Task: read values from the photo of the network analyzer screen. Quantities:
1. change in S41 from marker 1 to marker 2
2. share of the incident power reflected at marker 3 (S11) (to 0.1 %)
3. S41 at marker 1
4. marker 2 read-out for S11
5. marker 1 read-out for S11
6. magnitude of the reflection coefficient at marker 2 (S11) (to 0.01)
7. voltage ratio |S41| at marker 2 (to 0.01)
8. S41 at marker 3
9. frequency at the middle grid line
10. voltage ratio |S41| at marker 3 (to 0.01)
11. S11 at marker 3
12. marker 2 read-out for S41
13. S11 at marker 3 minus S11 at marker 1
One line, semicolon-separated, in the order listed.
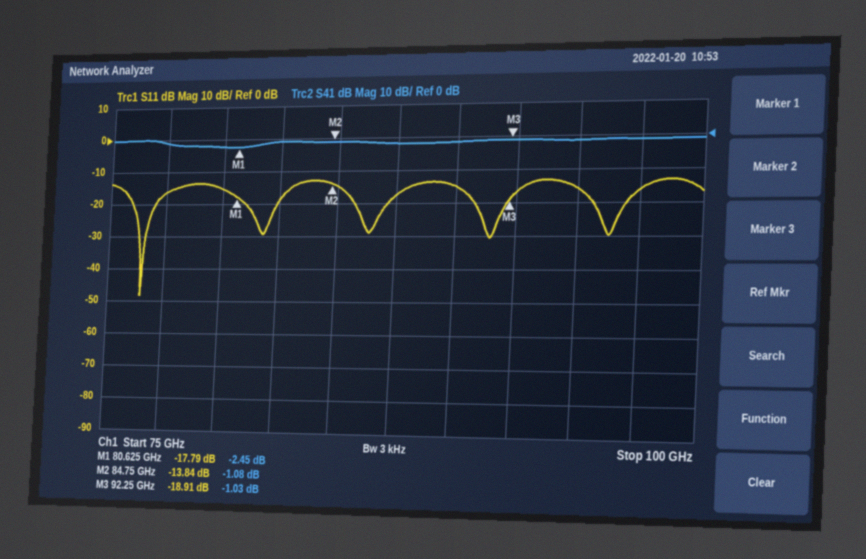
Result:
1.37 dB; 1.3 %; -2.45 dB; -13.84 dB; -17.79 dB; 0.20; 0.88; -1.03 dB; 87.5 GHz; 0.89; -18.91 dB; -1.08 dB; -1.12 dB
